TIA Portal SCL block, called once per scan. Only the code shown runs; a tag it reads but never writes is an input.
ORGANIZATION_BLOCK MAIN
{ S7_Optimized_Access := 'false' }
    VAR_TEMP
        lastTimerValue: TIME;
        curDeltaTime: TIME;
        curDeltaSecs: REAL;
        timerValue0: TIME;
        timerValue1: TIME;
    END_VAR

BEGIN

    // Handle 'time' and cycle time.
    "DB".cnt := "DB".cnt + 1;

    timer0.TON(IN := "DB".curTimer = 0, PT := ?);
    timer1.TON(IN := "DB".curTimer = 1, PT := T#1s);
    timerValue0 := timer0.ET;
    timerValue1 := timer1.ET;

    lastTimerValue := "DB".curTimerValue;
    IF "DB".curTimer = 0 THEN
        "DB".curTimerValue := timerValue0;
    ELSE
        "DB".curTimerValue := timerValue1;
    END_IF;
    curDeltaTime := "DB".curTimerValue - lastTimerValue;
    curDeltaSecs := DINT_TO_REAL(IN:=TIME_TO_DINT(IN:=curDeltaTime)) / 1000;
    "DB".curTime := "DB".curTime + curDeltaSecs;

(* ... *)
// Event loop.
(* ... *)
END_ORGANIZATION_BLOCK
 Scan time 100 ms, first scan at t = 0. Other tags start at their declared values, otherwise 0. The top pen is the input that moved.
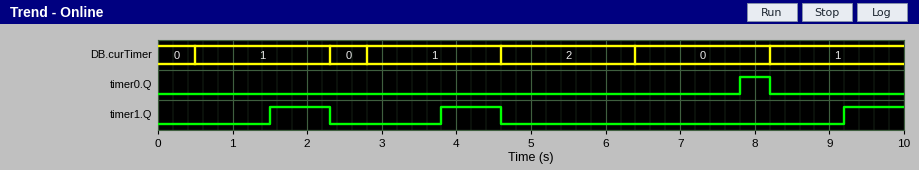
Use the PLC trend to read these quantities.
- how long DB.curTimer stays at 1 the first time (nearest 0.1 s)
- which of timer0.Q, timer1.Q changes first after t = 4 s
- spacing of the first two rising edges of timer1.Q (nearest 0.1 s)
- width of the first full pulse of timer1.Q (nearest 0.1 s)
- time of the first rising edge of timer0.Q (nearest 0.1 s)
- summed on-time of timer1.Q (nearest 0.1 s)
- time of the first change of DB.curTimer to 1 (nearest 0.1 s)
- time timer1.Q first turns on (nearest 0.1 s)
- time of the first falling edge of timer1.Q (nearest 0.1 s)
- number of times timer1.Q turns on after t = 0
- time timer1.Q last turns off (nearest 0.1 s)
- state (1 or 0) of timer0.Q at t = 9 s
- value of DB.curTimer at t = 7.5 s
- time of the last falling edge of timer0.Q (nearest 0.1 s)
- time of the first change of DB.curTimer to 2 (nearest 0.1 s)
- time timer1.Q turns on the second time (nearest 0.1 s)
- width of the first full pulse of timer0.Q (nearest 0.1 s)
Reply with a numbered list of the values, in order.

1. 1.8 s
2. timer1.Q
3. 2.3 s
4. 0.8 s
5. 7.8 s
6. 2.4 s
7. 0.5 s
8. 1.5 s
9. 2.3 s
10. 3
11. 4.6 s
12. 0
13. 0
14. 8.2 s
15. 4.6 s
16. 3.8 s
17. 0.4 s
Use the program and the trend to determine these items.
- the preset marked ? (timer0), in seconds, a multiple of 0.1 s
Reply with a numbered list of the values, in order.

1. 1.4 s
